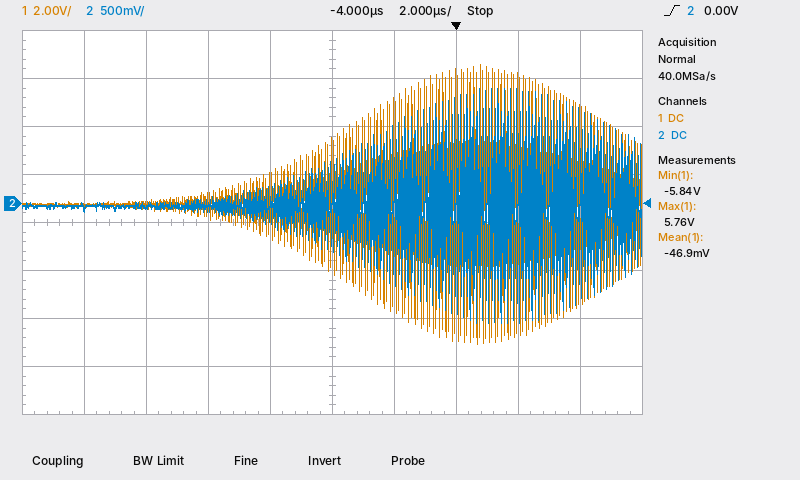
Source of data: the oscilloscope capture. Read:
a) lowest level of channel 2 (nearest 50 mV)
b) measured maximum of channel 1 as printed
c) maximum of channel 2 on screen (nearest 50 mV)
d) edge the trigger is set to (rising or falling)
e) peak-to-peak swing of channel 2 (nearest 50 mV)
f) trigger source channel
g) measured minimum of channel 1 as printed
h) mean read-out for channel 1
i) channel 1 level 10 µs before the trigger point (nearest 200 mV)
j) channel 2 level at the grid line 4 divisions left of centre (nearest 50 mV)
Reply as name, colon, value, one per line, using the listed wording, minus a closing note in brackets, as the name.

lowest level of channel 2: -1.25 V
measured maximum of channel 1 as printed: 5.76 V
maximum of channel 2 on screen: 1.20 V
edge the trigger is set to: rising
peak-to-peak swing of channel 2: 2.45 V
trigger source channel: channel 2
measured minimum of channel 1 as printed: -5.84 V
mean read-out for channel 1: -46.9 mV
channel 1 level 10 µs before the trigger point: 0.0 V
channel 2 level at the grid line 4 divisions left of centre: -50 mV
